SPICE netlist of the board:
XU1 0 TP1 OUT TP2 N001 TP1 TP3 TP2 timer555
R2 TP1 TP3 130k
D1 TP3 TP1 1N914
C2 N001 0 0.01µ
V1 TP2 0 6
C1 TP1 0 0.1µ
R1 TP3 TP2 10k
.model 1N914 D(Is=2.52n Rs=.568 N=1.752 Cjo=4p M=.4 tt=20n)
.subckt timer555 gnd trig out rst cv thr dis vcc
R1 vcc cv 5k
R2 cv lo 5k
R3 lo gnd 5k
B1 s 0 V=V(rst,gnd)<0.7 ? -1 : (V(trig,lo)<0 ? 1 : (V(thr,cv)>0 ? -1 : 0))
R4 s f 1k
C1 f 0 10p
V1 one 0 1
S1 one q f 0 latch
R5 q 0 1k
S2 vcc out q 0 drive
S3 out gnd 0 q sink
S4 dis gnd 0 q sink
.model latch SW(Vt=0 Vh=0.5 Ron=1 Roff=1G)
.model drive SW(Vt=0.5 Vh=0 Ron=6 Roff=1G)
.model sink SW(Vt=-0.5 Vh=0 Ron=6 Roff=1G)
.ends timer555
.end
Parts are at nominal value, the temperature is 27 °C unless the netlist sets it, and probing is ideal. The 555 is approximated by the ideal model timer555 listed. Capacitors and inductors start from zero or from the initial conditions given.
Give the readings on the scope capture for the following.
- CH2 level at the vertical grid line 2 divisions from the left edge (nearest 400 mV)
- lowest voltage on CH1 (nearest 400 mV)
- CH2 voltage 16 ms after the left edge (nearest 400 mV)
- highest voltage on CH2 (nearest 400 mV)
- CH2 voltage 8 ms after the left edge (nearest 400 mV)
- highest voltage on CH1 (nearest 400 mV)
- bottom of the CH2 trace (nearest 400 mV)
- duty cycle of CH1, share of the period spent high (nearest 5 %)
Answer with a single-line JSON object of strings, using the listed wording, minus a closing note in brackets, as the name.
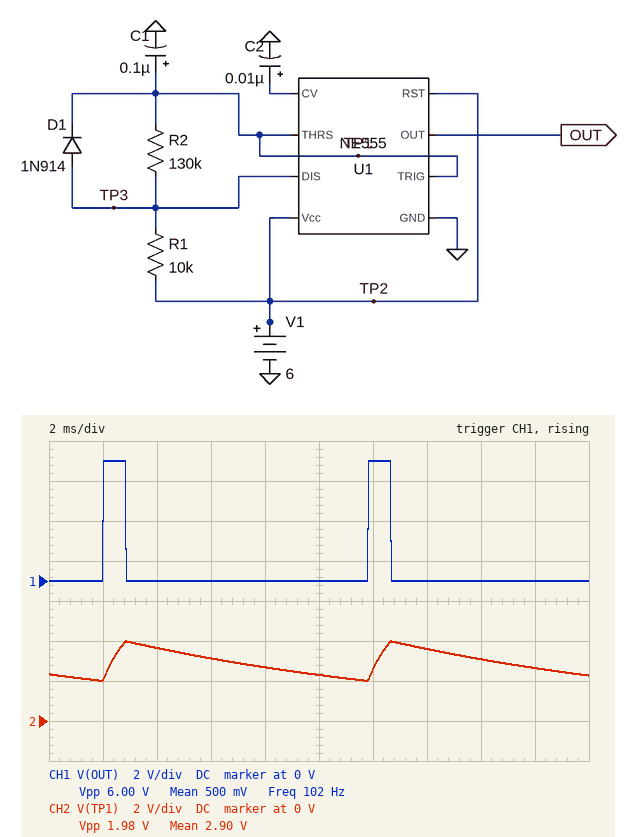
{"CH2 level at the vertical grid line 2 divisions from the left edge": "3.6 V", "lowest voltage on CH1": "0 V", "CH2 voltage 16 ms after the left edge": "3.2 V", "highest voltage on CH2": "4.0 V", "CH2 voltage 8 ms after the left edge": "2.8 V", "highest voltage on CH1": "6.0 V", "bottom of the CH2 trace": "2.0 V", "duty cycle of CH1, share of the period spent high": "10 %"}
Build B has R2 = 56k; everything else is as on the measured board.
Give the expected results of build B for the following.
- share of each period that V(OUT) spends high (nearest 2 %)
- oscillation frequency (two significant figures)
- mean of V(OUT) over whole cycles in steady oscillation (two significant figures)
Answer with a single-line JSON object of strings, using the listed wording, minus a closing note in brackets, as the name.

{"share of each period that V(OUT) spends high": "18 %", "oscillation frequency": "210 Hz", "mean of V(OUT) over whole cycles in steady oscillation": "1.1 V"}
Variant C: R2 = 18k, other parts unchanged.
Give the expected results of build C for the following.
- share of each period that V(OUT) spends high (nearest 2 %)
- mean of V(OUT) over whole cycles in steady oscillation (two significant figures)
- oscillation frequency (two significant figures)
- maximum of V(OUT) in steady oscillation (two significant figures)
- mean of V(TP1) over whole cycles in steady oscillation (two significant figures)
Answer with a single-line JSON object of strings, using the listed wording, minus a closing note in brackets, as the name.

{"share of each period that V(OUT) spends high": "40 %", "mean of V(OUT) over whole cycles in steady oscillation": "2.4 V", "oscillation frequency": "480 Hz", "maximum of V(OUT) in steady oscillation": "6.0 V", "mean of V(TP1) over whole cycles in steady oscillation": "3.0 V"}
